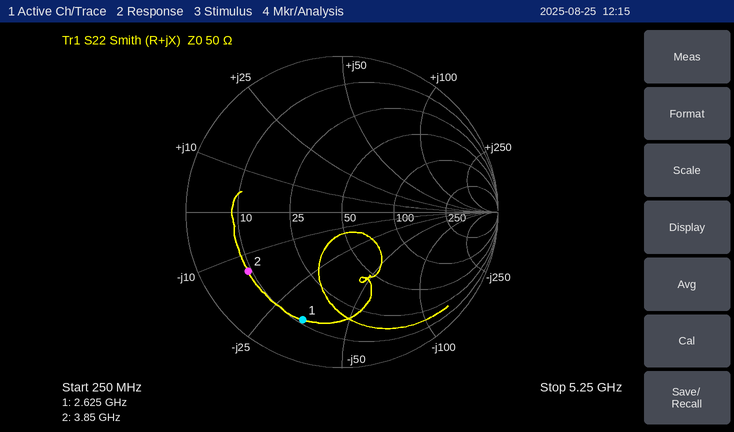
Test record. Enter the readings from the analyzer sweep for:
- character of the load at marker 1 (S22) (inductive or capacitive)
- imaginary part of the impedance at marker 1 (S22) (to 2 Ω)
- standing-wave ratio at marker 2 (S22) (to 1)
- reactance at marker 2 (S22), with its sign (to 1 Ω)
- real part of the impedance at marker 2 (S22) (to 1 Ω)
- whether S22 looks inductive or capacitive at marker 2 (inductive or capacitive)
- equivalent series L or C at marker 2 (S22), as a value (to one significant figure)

capacitive
-34 Ω
6
-14 Ω
9 Ω
capacitive
3 pF
